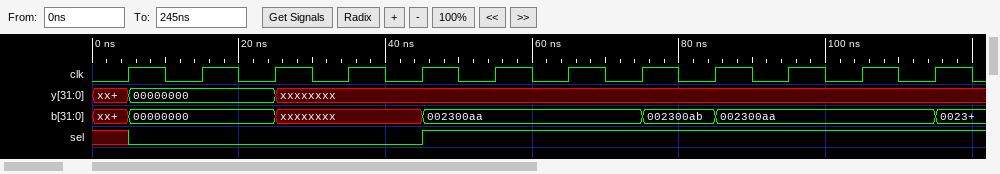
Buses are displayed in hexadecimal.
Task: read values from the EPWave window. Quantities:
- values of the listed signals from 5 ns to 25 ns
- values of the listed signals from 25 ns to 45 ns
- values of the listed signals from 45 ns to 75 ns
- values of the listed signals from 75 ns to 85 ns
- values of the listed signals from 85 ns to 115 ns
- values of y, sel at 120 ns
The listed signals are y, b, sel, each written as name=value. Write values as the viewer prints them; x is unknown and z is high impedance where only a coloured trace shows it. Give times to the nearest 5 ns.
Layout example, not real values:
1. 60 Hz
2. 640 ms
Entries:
1. y=00000000, b=00000000, sel=0
2. y=xxxxxxxx, b=xxxxxxxx, sel=0
3. y=xxxxxxxx, b=002300aa, sel=1
4. y=xxxxxxxx, b=002300ab, sel=1
5. y=xxxxxxxx, b=002300aa, sel=1
6. y=xxxxxxxx, sel=1
